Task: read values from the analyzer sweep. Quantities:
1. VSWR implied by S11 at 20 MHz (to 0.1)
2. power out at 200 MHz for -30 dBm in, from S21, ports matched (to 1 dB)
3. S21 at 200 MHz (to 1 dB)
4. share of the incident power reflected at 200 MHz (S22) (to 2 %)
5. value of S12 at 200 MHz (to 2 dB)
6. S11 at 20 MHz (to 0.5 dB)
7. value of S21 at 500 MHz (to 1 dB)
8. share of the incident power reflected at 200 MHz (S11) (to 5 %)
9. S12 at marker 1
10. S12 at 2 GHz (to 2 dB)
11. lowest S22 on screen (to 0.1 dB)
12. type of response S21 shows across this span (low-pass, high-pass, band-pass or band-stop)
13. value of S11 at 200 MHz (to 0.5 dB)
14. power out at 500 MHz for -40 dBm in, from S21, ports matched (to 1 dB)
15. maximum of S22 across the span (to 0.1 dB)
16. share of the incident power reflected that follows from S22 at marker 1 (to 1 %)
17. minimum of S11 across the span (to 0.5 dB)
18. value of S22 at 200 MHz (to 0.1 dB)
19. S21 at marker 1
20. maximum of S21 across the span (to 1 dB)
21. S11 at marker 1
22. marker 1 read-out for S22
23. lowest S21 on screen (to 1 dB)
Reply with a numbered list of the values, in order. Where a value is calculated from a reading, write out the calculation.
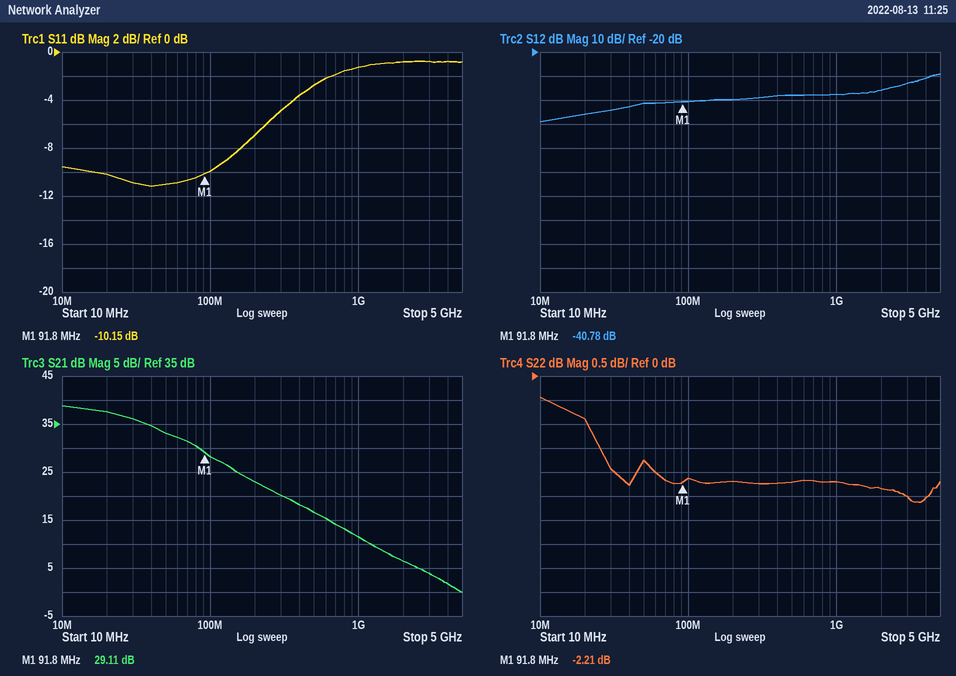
1. |Γ| = 10^(-10/20) = 0.3162; VSWR = (1 + 0.3162)/(1 − 0.3162) ≈ 1.9
2. -30 dBm + (23 dB) = -7 dBm
3. 23 dB
4. 10^(-2.2/10) ≈ 60 %
5. -40 dB
6. -10.0 dB
7. 17 dB
8. 10^(-7/10) ≈ 20 %
9. -40.78 dB
10. -36 dB
11. -2.6 dB
12. low-pass
13. -7.0 dB
14. -40 dBm + (17 dB) = -23 dBm
15. -0.4 dB
16. 10^(-2.21/10) ≈ 60 %
17. -11.0 dB
18. -2.2 dB
19. 29.11 dB
20. 39 dB
21. -10.15 dB
22. -2.21 dB
23. 0 dB
